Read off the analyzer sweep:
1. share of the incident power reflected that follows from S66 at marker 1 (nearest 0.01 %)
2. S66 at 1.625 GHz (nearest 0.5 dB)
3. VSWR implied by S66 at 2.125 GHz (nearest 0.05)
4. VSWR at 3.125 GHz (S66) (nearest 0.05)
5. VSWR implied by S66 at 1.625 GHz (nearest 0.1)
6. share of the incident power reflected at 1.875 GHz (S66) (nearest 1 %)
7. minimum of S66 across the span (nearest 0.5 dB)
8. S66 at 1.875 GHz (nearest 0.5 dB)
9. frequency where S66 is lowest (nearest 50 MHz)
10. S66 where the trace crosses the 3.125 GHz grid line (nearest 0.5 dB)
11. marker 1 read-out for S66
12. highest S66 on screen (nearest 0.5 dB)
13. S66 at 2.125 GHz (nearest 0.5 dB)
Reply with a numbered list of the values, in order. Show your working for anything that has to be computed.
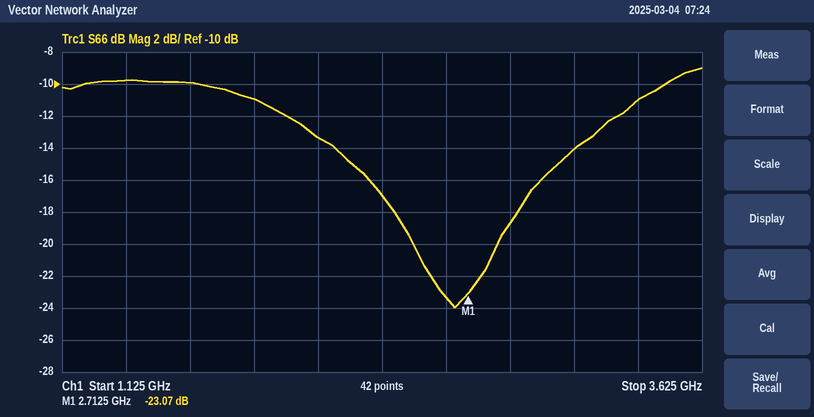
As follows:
1. 10^(-23.07/10) ≈ 0.49 %
2. -10.0 dB
3. |Γ| = 10^(-13.5/20) = 0.2113; VSWR = (1 + 0.2113)/(1 − 0.2113) ≈ 1.54, so 1.55 to the nearest 0.05
4. |Γ| = 10^(-14/20) = 0.1995; VSWR = (1 + 0.1995)/(1 − 0.1995) ≈ 1.50
5. |Γ| = 10^(-10/20) = 0.3162; VSWR = (1 + 0.3162)/(1 − 0.3162) ≈ 1.9
6. 10^(-11/10) ≈ 8 %
7. -24.0 dB
8. -11.0 dB
9. 2.65 GHz
10. -14.0 dB
11. -23.07 dB
12. -9.0 dB
13. -13.5 dB
